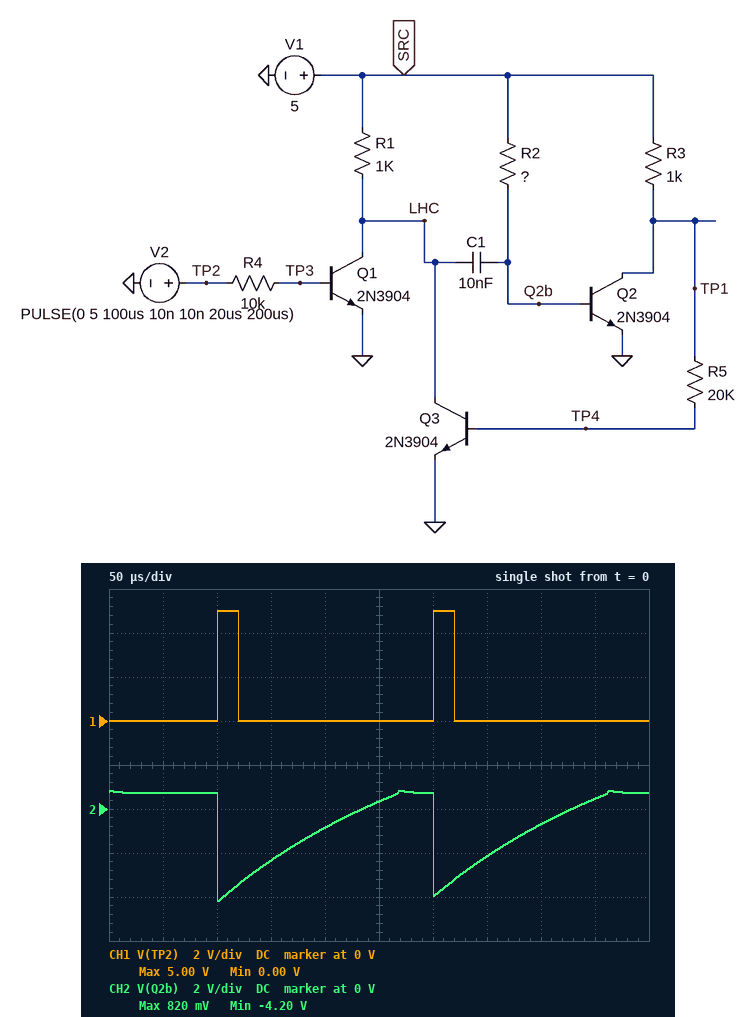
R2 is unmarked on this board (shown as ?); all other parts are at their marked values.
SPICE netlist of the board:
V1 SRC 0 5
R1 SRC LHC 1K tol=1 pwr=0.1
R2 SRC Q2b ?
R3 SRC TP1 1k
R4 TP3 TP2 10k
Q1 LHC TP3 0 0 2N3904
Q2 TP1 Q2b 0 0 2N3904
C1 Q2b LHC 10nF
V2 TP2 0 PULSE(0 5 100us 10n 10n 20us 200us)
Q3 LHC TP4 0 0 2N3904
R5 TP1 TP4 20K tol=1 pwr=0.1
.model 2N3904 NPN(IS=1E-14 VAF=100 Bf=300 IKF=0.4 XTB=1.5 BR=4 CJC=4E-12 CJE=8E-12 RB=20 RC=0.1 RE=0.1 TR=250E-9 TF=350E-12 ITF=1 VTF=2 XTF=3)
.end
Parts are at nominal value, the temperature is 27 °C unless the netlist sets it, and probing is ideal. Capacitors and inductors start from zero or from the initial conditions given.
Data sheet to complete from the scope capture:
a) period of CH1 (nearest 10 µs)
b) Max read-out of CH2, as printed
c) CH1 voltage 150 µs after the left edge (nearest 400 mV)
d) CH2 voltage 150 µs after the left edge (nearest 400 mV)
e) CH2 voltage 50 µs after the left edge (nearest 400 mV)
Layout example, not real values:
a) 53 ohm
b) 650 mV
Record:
a) 200 µs
b) 820 mV
c) 0 V
d) -2.4 V
e) 800 mV
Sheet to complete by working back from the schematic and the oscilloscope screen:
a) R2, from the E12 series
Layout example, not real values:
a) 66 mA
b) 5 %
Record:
a) 22 kΩ
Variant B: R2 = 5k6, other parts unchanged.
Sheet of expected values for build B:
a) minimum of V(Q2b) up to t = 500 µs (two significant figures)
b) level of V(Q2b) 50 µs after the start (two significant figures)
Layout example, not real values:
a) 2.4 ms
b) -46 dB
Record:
a) -4.1 V
b) 730 mV
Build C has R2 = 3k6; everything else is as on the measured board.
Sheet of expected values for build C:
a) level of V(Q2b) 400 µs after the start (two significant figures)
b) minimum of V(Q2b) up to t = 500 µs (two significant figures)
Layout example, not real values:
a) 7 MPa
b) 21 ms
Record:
a) 740 mV
b) -4.0 V
